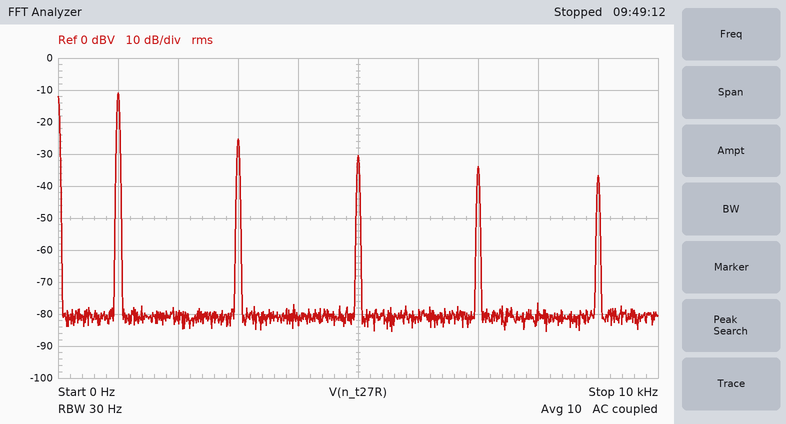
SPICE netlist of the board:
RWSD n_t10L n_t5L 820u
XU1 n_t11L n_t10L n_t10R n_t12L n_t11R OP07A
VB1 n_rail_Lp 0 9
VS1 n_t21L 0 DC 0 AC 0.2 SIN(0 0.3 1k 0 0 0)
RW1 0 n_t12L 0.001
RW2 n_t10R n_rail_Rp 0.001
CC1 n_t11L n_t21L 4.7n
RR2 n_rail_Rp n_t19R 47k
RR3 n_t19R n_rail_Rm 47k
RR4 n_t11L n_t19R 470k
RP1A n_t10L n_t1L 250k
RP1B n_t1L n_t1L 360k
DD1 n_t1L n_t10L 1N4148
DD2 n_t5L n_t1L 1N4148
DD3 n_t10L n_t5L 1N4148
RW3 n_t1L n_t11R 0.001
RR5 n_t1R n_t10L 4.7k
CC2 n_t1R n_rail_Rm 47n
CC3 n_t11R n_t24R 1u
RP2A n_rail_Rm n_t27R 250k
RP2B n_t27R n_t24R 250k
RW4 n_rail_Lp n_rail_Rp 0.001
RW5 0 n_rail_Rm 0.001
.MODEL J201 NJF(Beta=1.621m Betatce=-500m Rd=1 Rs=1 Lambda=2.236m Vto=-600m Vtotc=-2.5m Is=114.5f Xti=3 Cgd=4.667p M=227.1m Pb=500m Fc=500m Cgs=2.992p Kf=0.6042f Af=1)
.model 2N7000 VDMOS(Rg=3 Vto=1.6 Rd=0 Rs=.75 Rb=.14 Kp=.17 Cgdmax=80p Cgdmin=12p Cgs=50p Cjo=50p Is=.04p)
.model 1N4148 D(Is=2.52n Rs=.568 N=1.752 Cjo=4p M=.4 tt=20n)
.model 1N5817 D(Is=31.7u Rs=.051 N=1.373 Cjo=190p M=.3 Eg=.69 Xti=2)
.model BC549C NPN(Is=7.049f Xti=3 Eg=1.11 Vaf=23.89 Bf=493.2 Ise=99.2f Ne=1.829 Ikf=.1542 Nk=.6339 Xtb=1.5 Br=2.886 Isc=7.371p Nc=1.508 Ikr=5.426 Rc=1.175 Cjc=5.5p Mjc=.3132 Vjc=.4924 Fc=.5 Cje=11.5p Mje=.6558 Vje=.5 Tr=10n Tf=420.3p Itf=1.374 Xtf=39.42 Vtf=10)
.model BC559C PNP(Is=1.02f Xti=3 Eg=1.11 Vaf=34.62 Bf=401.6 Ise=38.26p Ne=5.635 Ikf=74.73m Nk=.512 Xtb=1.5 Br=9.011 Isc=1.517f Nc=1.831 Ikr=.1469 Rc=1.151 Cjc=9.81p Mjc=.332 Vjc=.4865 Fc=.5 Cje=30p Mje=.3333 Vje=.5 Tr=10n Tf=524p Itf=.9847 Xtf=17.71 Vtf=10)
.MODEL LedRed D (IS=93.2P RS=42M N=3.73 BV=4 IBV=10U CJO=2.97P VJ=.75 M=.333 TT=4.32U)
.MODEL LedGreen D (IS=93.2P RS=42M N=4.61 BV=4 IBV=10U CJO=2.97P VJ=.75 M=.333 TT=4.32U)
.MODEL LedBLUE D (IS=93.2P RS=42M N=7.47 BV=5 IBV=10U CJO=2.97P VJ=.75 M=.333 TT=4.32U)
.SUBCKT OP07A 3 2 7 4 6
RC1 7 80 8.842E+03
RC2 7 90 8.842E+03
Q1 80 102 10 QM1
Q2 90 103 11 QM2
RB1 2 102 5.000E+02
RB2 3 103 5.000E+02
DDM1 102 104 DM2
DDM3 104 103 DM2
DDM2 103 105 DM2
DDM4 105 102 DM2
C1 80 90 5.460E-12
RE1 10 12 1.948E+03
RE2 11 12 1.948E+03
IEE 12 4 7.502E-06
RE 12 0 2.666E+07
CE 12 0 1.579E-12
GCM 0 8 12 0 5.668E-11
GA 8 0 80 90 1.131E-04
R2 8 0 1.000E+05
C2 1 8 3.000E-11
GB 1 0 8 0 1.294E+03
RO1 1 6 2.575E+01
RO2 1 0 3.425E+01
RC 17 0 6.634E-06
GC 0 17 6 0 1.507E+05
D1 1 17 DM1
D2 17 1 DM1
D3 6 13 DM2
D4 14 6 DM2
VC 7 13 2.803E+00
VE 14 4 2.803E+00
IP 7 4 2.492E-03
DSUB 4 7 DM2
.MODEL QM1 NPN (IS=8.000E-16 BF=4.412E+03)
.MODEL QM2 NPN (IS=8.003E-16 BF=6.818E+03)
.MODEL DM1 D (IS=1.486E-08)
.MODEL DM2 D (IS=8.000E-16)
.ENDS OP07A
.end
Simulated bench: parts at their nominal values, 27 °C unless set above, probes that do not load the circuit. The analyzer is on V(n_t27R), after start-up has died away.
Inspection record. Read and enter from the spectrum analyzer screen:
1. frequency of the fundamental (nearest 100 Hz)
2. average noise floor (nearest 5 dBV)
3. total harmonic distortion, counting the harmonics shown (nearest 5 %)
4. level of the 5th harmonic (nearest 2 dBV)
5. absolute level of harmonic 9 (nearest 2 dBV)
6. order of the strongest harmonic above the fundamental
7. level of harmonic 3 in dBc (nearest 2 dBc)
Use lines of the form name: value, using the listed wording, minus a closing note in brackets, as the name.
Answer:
frequency of the fundamental: 1.0 kHz
average noise floor: -80 dBV
total harmonic distortion, counting the harmonics shown: 25 %
level of the 5th harmonic: -30 dBV
absolute level of harmonic 9: -36 dBV
order of the strongest harmonic above the fundamental: 3
level of harmonic 3 in dBc: -14 dBc
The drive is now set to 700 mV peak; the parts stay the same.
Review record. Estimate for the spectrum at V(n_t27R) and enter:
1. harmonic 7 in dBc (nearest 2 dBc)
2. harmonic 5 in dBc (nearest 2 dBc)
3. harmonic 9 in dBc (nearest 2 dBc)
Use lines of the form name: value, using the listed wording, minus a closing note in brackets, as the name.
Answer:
harmonic 7 in dBc: -26 dBc
harmonic 5 in dBc: -22 dBc
harmonic 9 in dBc: -28 dBc
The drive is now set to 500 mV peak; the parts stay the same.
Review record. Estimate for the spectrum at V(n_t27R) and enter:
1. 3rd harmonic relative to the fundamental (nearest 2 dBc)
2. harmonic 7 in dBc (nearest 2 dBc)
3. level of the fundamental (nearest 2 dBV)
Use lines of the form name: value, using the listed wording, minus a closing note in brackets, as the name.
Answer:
3rd harmonic relative to the fundamental: -16 dBc
harmonic 7 in dBc: -24 dBc
level of the fundamental: -8 dBV
